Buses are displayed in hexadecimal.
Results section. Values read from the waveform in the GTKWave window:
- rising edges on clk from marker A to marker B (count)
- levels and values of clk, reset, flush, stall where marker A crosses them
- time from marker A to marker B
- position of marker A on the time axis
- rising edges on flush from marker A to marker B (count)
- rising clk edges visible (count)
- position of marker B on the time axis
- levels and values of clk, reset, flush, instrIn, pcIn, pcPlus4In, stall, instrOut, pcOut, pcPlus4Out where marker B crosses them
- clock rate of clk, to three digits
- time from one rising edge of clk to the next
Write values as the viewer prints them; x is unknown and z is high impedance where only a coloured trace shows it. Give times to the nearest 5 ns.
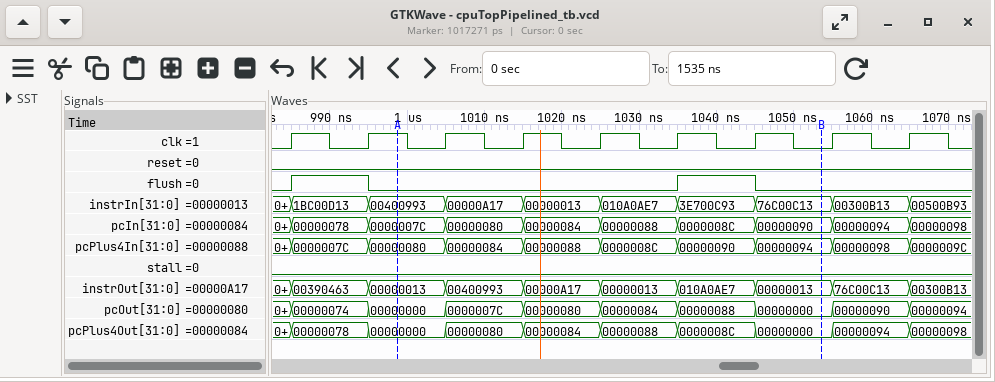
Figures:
5
clk=1, reset=0, flush=0, stall=0
55 ns
1000 ns
1
9
1055 ns
clk=0, reset=0, flush=0, instrIn=76C00C13, pcIn=00000090, pcPlus4In=00000094, stall=0, instrOut=00000013, pcOut=00000000, pcPlus4Out=00000000
100 MHz
10 ns
